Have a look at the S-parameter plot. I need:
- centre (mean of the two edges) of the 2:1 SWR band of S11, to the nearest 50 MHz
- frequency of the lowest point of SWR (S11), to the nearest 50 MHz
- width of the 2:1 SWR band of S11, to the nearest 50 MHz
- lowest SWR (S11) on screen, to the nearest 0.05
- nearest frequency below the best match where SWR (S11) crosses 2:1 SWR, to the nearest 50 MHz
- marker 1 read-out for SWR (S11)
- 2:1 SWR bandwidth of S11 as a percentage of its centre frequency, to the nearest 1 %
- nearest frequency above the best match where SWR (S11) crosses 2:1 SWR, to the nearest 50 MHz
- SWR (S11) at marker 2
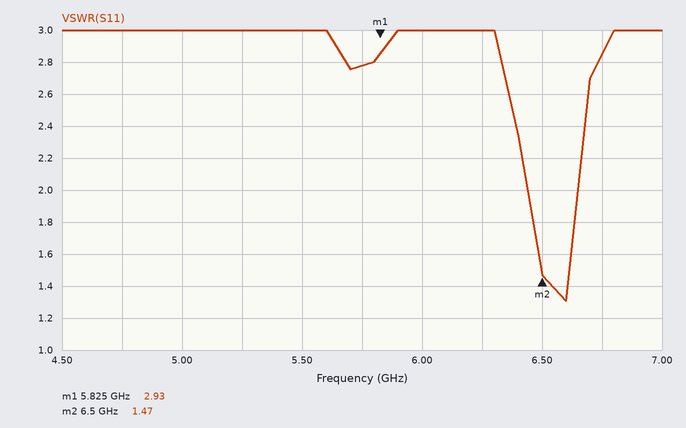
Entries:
6.55 GHz
6.60 GHz
200 MHz
1.30
6.45 GHz
2.93
3 %
6.65 GHz
1.47
